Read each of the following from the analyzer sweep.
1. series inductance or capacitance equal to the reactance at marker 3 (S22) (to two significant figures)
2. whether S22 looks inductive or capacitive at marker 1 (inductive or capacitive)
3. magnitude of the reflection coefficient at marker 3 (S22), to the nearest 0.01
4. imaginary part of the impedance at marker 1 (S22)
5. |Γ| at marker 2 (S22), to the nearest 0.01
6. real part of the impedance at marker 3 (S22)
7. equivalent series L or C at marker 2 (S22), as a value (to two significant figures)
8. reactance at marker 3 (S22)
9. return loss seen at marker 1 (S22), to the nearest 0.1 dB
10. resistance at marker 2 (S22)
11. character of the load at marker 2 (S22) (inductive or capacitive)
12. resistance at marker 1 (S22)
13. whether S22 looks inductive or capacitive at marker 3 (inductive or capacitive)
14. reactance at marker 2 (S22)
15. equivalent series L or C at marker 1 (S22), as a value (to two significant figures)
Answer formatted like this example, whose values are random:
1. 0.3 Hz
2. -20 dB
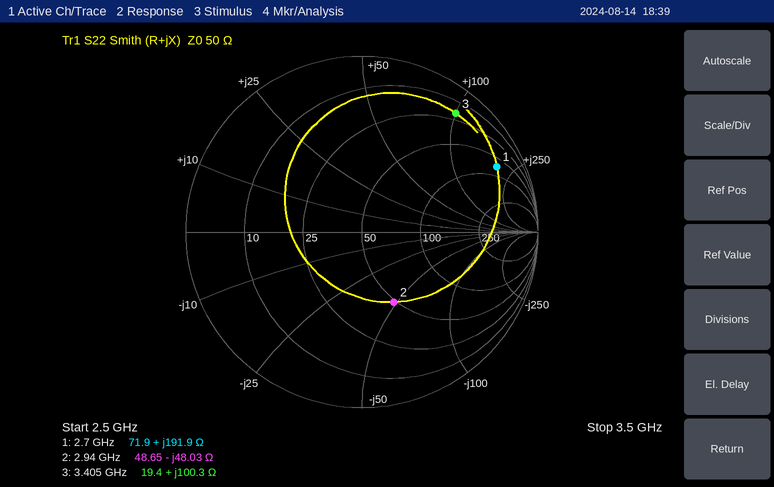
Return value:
1. 4.7 nH
2. inductive
3. 0.86
4. +191.9 Ω
5. 0.44
6. 19.4 Ω
7. 1.1 pF
8. +100.3 Ω
9. 1.4 dB
10. 48.65 Ω
11. capacitive
12. 71.9 Ω
13. inductive
14. -48.03 Ω
15. 11 nH
